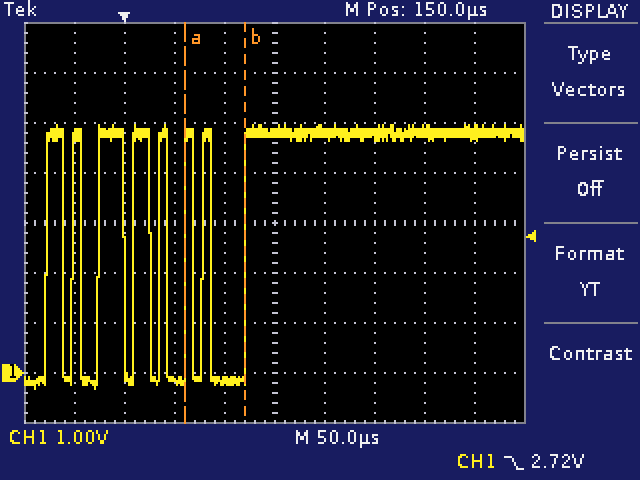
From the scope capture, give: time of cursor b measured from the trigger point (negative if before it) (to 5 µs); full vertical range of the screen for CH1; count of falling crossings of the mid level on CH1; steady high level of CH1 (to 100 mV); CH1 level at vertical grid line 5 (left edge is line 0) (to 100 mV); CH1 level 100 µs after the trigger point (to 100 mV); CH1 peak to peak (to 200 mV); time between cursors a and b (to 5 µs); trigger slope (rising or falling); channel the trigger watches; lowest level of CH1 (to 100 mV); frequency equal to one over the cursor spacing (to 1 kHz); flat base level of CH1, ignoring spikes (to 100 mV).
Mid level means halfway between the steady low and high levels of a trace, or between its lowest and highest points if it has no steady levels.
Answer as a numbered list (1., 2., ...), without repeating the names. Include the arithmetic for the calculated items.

1. +120 µs
2. 8 V
3. 7
4. 4.8 V
5. 4.8 V
6. -200 mV
7. 5.2 V
8. 60 µs
9. falling
10. CH1
11. -300 mV
12. 1 / 60 µs ≈ 17 kHz
13. -200 mV
